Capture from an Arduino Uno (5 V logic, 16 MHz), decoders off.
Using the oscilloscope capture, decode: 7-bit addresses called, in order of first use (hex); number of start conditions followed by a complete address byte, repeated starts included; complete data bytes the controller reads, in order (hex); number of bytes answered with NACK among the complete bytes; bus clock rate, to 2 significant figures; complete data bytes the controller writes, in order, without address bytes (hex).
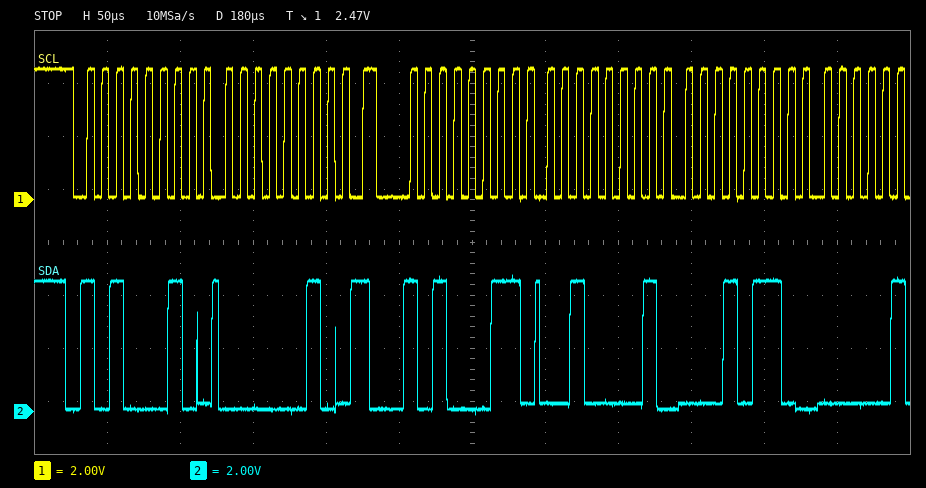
0x51
2
21 16
0
100 kHz
02
